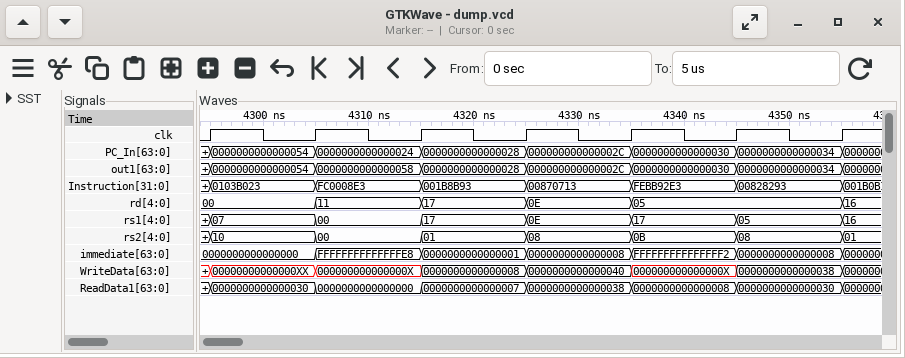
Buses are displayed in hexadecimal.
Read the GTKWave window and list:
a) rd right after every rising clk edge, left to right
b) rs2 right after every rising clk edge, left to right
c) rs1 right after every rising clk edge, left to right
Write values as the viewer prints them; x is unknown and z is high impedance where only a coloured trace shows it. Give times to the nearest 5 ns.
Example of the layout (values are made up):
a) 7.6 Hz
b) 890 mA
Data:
a) 00, 11, 17, 0E, 05, 05, 16
b) 10, 00, 01, 08, 0B, 08, 01
c) 07, 00, 17, 0E, 17, 05, 16
